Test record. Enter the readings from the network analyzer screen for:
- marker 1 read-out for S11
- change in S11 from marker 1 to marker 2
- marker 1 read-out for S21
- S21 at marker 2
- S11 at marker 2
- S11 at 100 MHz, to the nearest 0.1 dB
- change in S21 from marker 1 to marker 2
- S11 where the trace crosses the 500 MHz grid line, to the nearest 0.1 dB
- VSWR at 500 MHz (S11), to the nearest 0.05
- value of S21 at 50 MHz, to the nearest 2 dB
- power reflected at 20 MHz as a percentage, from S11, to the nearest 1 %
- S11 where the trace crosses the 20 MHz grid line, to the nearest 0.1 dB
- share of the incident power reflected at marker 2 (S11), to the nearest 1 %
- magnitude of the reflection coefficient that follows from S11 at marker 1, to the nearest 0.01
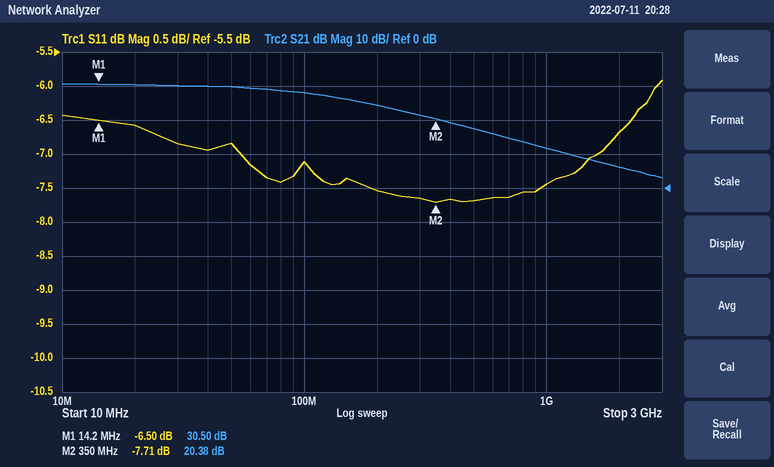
-6.50 dB
-1.21 dB
30.50 dB
20.38 dB
-7.71 dB
-7.1 dB
-10.12 dB
-7.7 dB
2.40
30 dB
22 %
-6.6 dB
17 %
0.47
